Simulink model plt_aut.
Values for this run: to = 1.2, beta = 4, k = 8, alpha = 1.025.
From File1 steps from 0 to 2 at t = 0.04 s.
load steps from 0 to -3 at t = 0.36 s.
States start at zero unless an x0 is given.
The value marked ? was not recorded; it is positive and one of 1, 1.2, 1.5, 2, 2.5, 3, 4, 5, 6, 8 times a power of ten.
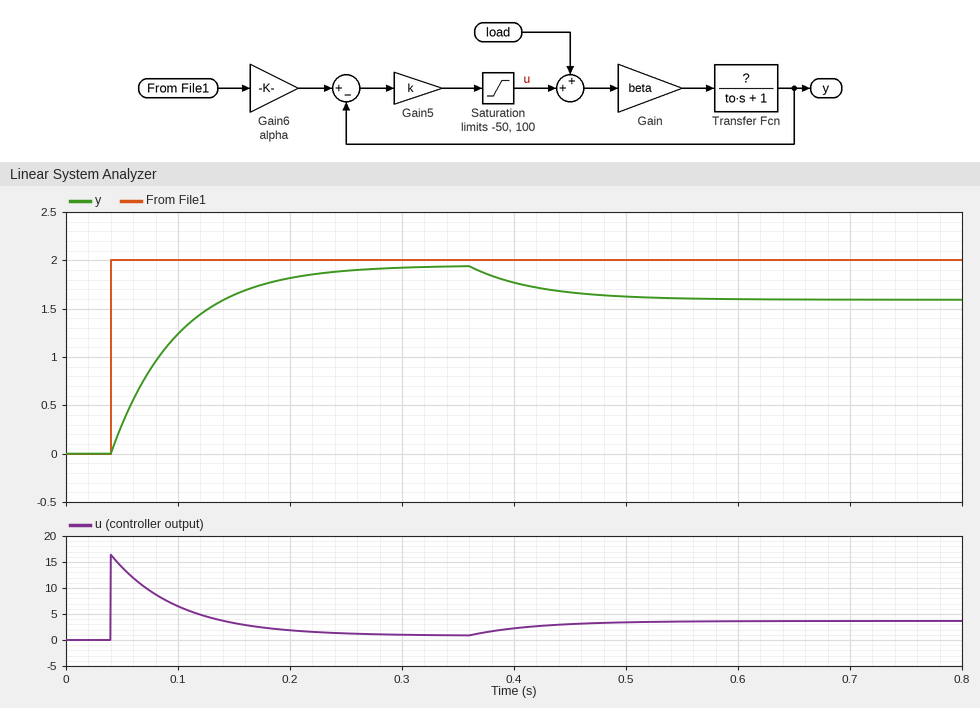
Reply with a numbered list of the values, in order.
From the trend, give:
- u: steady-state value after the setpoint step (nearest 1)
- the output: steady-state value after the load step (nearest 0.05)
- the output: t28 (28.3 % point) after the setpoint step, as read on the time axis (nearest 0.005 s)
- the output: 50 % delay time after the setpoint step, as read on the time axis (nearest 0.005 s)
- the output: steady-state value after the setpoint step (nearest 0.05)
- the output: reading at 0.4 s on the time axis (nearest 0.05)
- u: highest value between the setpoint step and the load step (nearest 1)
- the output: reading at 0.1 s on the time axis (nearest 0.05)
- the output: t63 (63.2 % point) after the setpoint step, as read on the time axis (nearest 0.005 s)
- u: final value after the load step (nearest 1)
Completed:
1. 1
2. 1.60
3. 0.060 s
4. 0.080 s
5. 1.95
6. 1.75
7. 16
8. 1.25
9. 0.100 s
10. 4
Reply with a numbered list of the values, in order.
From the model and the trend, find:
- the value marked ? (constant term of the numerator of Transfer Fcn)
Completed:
1. 0.6
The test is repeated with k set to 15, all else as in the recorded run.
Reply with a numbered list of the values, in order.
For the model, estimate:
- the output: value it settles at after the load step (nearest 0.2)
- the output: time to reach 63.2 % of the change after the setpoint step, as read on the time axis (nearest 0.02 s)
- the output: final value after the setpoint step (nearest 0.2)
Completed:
1. 1.8
2. 0.08 s
3. 2.0
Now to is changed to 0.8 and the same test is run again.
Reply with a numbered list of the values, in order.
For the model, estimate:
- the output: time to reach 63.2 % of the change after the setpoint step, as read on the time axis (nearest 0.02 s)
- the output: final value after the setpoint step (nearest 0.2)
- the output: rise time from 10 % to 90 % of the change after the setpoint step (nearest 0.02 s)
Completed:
1. 0.08 s
2. 2.0
3. 0.08 s
